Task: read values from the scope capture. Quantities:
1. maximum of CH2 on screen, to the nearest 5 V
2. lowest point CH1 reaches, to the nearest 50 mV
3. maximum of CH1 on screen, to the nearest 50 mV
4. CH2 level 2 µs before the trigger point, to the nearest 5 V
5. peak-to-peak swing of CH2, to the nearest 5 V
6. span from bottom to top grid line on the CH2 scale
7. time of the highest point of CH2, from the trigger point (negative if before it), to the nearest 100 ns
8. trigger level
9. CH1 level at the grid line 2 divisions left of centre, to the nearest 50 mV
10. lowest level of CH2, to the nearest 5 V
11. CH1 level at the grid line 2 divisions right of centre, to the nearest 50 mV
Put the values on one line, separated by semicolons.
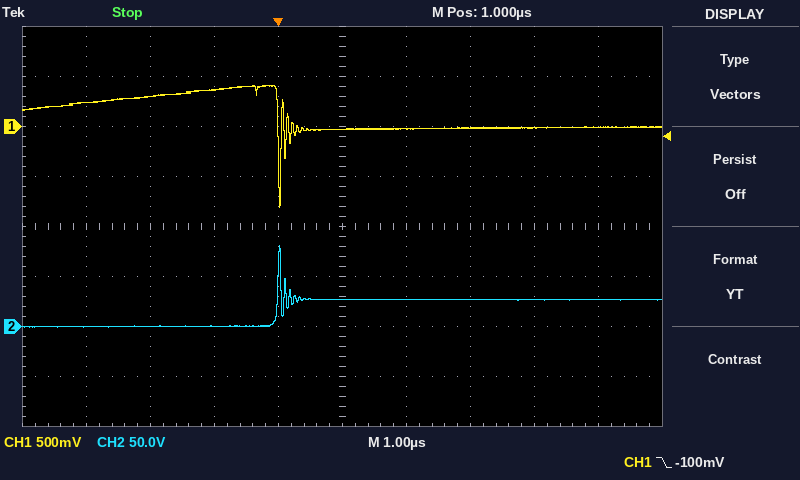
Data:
80 V; -800 mV; 400 mV; 0 V; 80 V; 400 V; 0.0 µs; -100 mV; 350 mV; 0 V; 0 mV
